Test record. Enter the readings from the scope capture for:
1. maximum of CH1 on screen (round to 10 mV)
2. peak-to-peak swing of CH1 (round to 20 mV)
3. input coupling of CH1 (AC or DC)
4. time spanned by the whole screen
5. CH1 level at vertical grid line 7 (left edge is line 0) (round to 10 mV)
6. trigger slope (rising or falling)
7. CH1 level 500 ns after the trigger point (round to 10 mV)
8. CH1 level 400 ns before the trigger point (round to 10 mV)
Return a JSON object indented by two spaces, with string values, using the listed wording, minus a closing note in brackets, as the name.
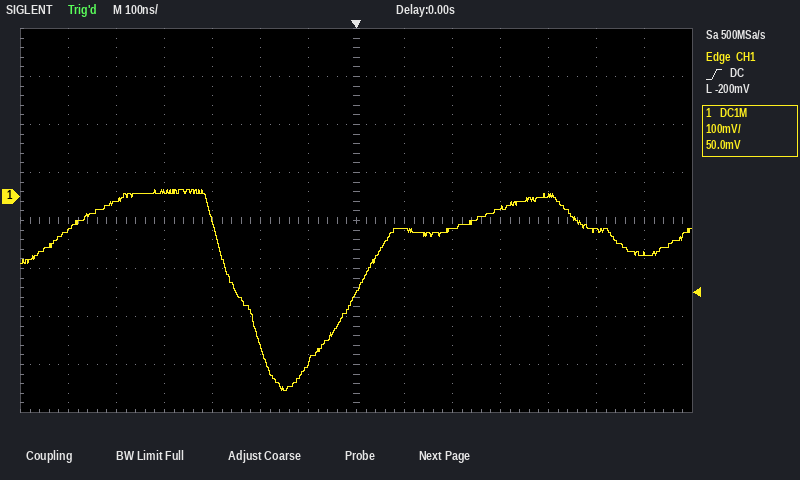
{
  "maximum of CH1 on screen": "10 mV",
  "peak-to-peak swing of CH1": "420 mV",
  "input coupling of CH1": "DC",
  "time spanned by the whole screen": "1.4 µs",
  "CH1 level at vertical grid line 7 (left edge is line 0)": "-200 mV",
  "trigger slope": "rising",
  "CH1 level 500 ns after the trigger point": "-70 mV",
  "CH1 level 400 ns before the trigger point": "10 mV"
}
